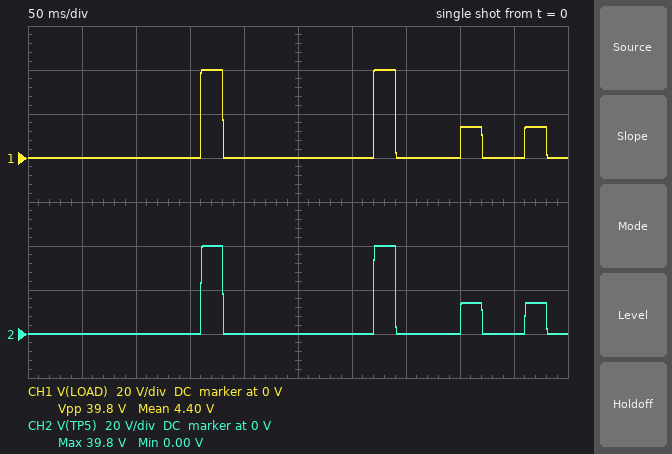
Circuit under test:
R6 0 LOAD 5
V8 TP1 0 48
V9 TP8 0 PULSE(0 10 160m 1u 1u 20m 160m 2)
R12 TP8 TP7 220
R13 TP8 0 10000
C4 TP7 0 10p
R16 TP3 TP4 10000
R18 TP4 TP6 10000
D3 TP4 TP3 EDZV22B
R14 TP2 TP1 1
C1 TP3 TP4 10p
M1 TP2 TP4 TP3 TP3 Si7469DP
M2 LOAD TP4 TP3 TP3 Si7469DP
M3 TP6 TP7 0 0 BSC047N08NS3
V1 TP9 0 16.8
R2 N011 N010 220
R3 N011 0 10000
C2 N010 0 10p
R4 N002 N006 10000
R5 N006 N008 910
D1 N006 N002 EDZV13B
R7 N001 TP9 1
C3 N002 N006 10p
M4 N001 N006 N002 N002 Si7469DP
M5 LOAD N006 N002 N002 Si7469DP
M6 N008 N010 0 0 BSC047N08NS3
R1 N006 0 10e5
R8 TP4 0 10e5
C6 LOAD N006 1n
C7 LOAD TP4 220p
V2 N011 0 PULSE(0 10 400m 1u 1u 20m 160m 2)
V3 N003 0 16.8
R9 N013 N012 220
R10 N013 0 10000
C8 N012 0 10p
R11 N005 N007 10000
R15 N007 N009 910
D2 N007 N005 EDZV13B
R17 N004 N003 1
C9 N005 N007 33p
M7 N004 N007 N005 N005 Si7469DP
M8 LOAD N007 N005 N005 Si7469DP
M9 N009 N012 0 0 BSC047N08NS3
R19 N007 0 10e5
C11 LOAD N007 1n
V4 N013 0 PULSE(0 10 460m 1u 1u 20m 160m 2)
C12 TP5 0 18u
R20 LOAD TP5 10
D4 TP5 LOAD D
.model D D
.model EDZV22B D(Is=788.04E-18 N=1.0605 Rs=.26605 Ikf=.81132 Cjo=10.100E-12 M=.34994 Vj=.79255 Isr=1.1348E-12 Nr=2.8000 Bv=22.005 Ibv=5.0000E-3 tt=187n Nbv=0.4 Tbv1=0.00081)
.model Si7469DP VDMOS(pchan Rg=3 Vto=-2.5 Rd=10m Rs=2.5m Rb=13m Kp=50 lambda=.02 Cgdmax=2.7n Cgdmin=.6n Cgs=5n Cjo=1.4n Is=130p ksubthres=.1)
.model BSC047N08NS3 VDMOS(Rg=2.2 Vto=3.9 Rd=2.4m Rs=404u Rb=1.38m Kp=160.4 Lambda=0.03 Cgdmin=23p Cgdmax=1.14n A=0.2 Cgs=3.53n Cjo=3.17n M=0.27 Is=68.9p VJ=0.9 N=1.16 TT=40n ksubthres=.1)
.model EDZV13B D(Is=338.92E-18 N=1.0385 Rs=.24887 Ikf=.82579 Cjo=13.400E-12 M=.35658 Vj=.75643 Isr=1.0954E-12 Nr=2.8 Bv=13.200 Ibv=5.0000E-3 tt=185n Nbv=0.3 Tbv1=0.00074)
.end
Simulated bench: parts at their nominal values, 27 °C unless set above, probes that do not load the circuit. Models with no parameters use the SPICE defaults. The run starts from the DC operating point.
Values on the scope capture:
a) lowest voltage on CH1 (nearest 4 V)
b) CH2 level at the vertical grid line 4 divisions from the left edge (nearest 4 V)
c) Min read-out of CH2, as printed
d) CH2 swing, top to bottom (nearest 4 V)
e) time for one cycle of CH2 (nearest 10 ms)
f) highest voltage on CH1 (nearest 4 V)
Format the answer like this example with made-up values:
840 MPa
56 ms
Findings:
0 V
0 V
0.00 V
40 V
160 ms
40 V
